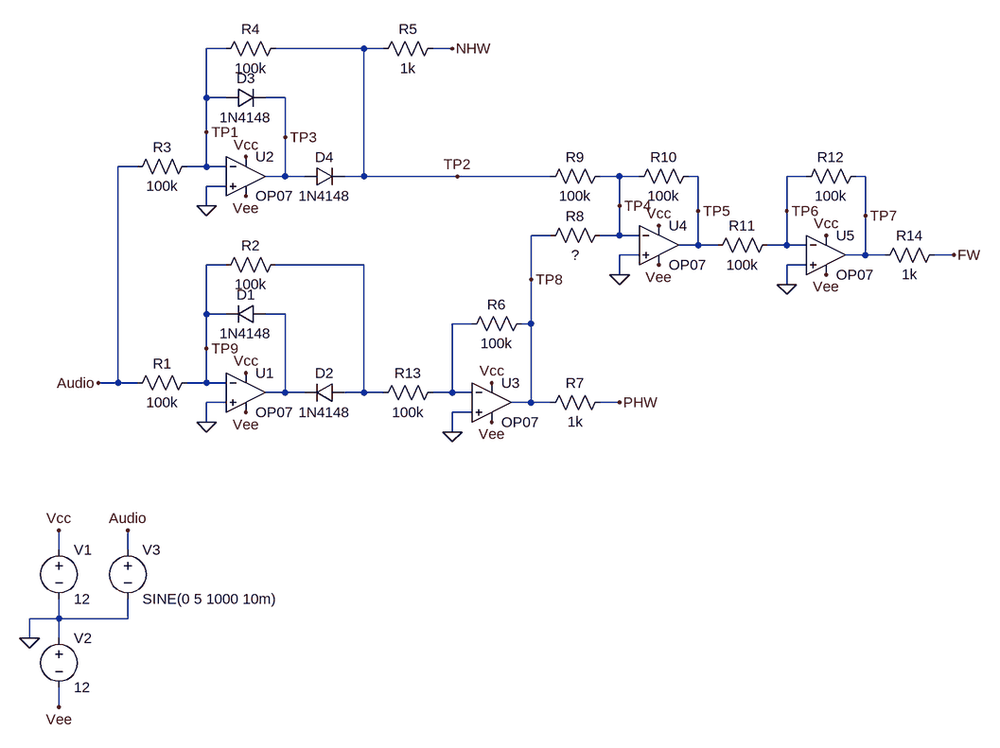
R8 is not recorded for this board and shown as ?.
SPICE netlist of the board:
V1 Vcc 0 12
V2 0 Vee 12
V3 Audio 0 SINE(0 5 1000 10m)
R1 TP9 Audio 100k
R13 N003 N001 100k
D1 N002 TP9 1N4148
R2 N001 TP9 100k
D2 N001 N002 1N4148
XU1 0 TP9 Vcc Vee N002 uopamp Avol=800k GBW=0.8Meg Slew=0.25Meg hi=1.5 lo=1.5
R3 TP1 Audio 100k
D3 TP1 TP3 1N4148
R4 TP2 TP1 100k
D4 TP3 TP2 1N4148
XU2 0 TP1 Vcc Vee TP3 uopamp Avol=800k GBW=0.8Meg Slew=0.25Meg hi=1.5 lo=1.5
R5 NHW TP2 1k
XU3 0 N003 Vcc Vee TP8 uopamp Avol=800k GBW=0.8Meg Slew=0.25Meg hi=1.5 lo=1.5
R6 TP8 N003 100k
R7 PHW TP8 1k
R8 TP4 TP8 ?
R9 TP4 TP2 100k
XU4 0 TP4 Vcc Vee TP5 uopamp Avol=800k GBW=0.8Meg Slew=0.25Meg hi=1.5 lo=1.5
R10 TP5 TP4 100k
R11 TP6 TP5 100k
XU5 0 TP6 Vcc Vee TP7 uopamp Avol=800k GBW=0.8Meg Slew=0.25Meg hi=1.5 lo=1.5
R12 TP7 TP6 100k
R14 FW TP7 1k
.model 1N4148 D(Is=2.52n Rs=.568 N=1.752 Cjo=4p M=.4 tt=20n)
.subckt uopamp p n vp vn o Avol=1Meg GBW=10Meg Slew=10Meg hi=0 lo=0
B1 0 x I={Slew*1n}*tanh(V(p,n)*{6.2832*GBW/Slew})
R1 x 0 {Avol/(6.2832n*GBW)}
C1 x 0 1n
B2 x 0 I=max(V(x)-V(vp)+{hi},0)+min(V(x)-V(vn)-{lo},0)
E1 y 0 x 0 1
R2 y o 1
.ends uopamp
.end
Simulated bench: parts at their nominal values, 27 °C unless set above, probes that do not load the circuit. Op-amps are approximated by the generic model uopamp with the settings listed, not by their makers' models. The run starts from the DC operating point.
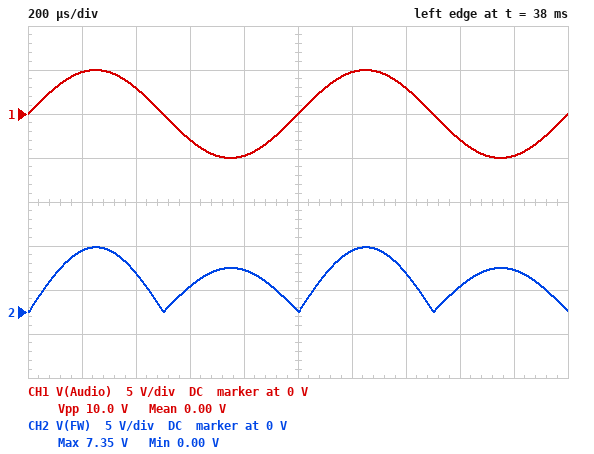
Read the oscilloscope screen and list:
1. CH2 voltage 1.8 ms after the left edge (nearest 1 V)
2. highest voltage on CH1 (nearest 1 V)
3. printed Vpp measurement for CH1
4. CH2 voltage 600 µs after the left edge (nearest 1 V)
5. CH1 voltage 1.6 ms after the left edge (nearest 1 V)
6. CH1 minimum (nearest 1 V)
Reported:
5 V
5 V
10.0 V
3 V
-3 V
-5 V
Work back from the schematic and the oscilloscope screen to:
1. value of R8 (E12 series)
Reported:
68 kΩ
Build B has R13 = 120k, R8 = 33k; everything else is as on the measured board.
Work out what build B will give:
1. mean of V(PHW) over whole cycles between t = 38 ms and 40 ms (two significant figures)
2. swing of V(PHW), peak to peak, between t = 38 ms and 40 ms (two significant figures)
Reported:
1.3 V
4.2 V
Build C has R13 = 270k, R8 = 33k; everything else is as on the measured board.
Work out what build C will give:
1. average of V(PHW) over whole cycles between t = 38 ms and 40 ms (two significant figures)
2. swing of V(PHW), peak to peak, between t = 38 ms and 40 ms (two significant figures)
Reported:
590 mV
1.9 V
